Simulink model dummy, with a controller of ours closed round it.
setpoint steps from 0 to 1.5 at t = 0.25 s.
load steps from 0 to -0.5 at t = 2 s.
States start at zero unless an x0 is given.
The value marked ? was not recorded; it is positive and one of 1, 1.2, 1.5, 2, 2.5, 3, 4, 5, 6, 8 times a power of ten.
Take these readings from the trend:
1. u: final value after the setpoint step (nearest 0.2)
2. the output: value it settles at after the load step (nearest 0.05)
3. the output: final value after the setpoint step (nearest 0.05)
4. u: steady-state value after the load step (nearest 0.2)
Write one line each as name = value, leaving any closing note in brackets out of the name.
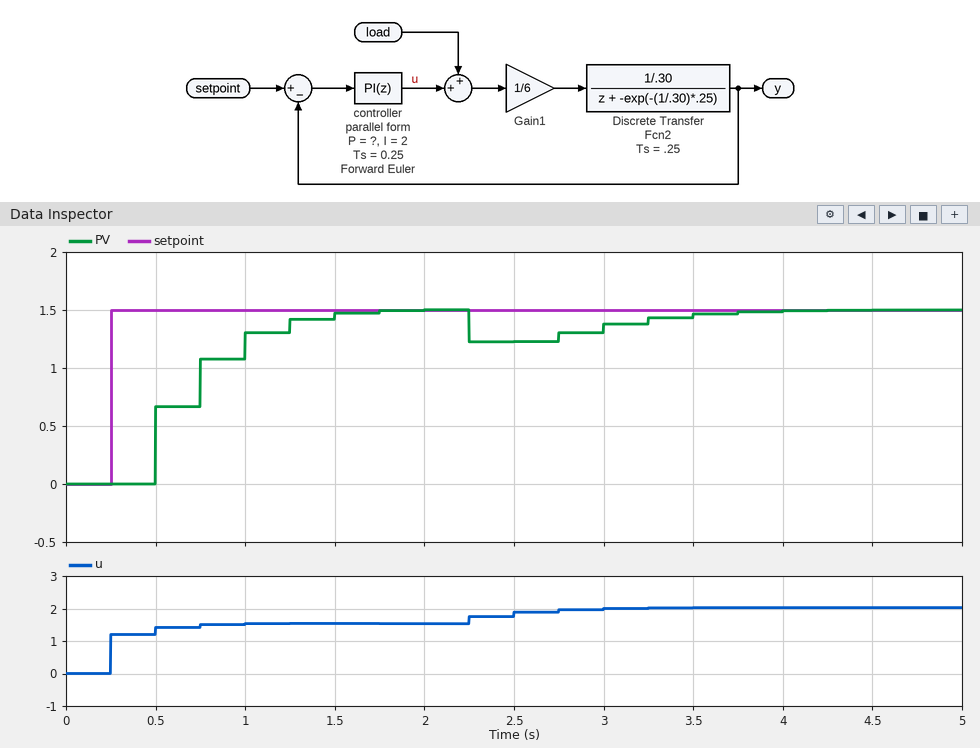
u: final value after the setpoint step = 1.6
the output: value it settles at after the load step = 1.50
the output: final value after the setpoint step = 1.50
u: steady-state value after the load step = 2.0
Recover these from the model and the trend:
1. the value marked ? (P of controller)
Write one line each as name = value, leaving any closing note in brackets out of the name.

the value marked ? = 0.8
